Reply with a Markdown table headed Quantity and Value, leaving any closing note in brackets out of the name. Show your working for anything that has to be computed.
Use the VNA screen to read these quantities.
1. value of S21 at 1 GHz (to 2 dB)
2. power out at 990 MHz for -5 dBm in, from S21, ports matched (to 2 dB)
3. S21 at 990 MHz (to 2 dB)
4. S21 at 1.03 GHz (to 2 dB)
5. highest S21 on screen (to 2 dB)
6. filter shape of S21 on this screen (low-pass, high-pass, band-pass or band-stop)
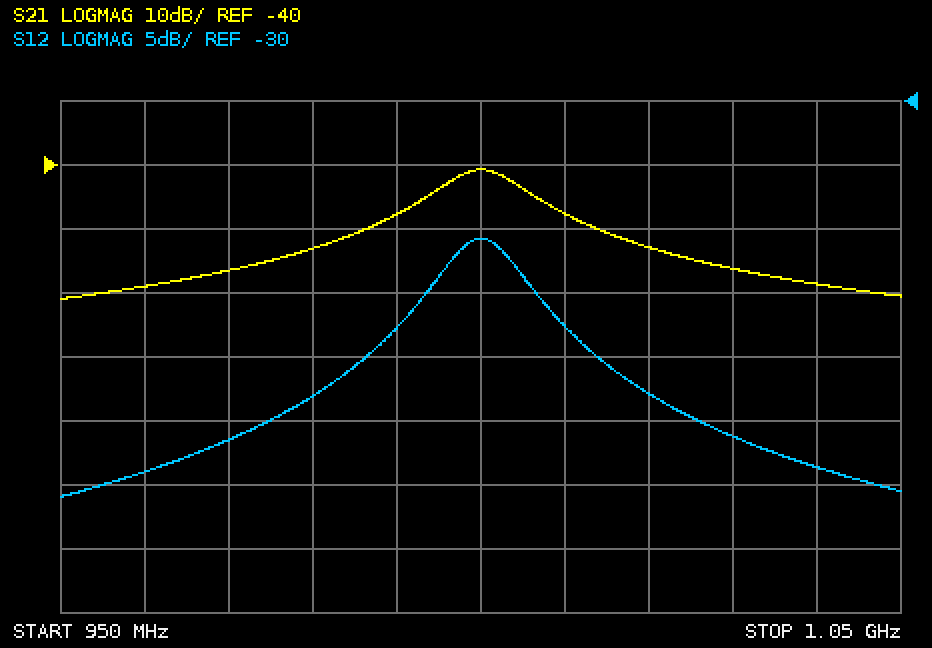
| Quantity | Value |
|---|---|
| value of S21 at 1 GHz | -40 dB |
| power out at 990 MHz for -5 dBm in, from S21, ports matched | -5 dBm + (-48 dB) = -52 dBm |
| S21 at 990 MHz | -48 dB |
| S21 at 1.03 GHz | -56 dB |
| highest S21 on screen | -40 dB |
| filter shape of S21 on this screen | band-pass |
